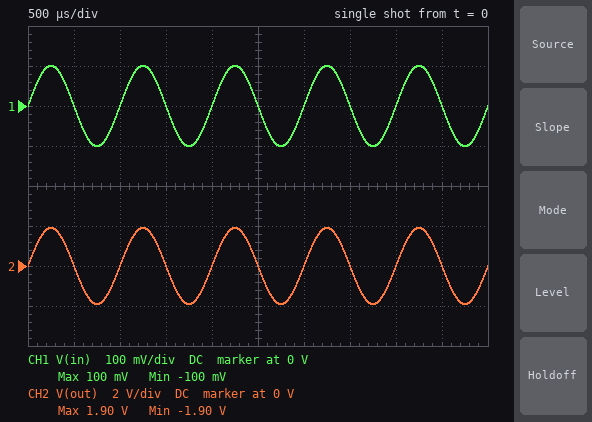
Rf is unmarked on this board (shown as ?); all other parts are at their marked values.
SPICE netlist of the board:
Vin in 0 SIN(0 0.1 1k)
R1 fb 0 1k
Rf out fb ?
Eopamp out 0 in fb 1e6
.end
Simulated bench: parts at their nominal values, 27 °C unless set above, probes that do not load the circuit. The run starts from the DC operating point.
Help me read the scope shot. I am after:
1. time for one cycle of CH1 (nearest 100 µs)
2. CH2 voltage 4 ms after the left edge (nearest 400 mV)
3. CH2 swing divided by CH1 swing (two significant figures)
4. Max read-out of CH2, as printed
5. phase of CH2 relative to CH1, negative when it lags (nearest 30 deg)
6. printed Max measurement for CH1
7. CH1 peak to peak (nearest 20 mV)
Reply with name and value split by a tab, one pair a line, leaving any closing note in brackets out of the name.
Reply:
time for one cycle of CH1	1.0 ms
CH2 voltage 4 ms after the left edge	0 V
CH2 swing divided by CH1 swing	19
Max read-out of CH2, as printed	1.90 V
phase of CH2 relative to CH1, negative when it lags	0 deg
printed Max measurement for CH1	100 mV
CH1 peak to peak	200 mV
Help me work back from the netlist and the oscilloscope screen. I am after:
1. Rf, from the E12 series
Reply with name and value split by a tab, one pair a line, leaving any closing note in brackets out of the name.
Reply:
Rf, from the E12 series	18 kΩ
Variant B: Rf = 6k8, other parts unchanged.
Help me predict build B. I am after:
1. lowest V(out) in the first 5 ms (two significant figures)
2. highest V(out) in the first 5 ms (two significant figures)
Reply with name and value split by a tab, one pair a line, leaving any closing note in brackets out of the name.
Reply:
lowest V(out) in the first 5 ms	-780 mV
highest V(out) in the first 5 ms	780 mV
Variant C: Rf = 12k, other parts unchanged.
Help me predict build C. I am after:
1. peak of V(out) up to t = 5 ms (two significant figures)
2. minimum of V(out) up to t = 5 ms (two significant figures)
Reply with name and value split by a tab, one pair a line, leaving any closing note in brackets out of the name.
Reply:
peak of V(out) up to t = 5 ms	1.3 V
minimum of V(out) up to t = 5 ms	-1.3 V
